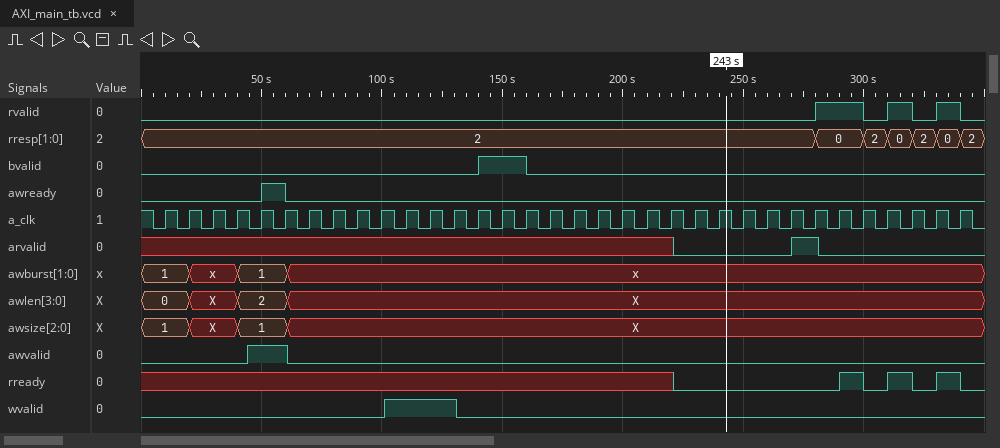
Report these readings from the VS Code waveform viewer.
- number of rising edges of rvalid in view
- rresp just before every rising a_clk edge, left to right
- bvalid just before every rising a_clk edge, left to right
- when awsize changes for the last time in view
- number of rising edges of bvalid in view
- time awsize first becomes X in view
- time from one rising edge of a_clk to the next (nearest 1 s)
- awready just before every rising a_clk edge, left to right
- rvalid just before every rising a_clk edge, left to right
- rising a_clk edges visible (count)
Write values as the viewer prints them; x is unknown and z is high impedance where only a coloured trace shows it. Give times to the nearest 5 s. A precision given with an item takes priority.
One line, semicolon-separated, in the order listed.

3; 2, 2, 2, 2, 2, 2, 2, 2, 2, 2, 2, 2, 2, 2, 2, 2, 2, 2, 2, 2, 2, 2, 2, 2, 2, 2, 2, 2, 0, 0, 2, 0, 2, 0; 0 0 0 0 0 0 0 0 0 0 0 0 0 0 1 1 0 0 0 0 0 0 0 0 0 0 0 0 0 0 0 0 0 0; 60 s; 1; 20 s; 10 s; 0 0 0 0 0 1 0 0 0 0 0 0 0 0 0 0 0 0 0 0 0 0 0 0 0 0 0 0 0 0 0 0 0 0; 0 0 0 0 0 0 0 0 0 0 0 0 0 0 0 0 0 0 0 0 0 0 0 0 0 0 0 0 1 1 0 1 0 1; 34
